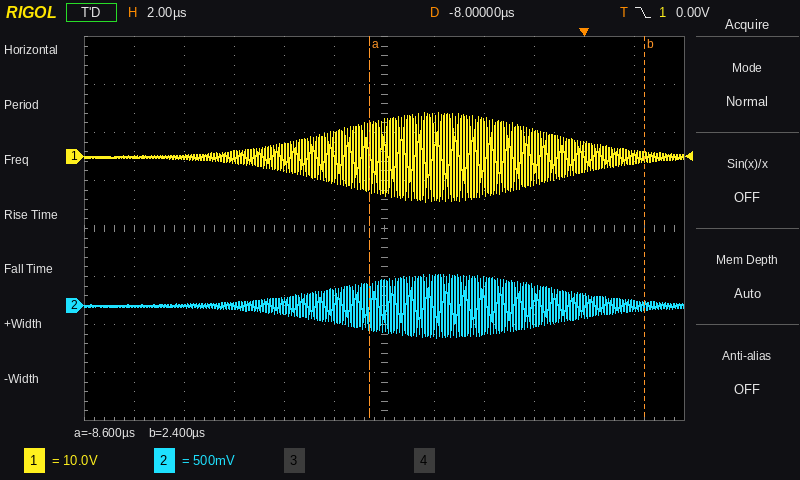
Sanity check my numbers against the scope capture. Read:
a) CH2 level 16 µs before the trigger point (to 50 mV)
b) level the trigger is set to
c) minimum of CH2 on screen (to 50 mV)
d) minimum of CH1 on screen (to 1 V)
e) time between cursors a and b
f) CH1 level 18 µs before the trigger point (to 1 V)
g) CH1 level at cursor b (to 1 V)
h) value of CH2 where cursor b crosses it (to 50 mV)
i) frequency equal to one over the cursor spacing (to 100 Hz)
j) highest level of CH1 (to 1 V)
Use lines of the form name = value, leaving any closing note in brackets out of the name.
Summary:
CH2 level 16 µs before the trigger point = 0 mV
level the trigger is set to = 0.00 V
minimum of CH2 on screen = -350 mV
minimum of CH1 on screen = -9 V
time between cursors a and b = 11.0 µs
CH1 level 18 µs before the trigger point = 0 V
CH1 level at cursor b = 0 V
value of CH2 where cursor b crosses it = 0 mV
frequency equal to one over the cursor spacing = 90.9 kHz
highest level of CH1 = 9 V
